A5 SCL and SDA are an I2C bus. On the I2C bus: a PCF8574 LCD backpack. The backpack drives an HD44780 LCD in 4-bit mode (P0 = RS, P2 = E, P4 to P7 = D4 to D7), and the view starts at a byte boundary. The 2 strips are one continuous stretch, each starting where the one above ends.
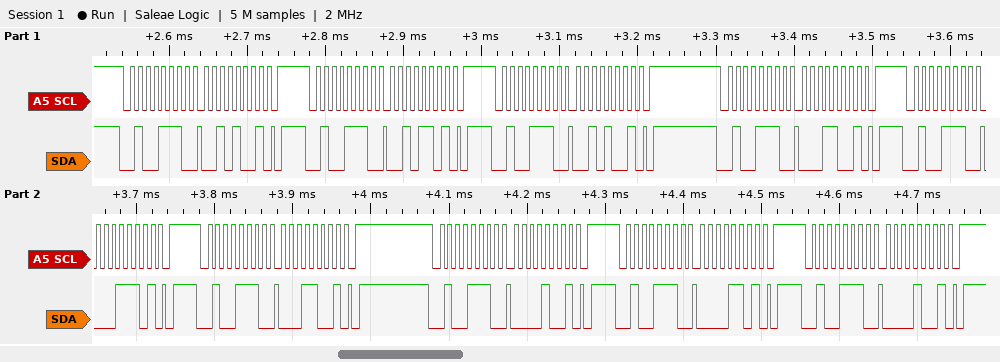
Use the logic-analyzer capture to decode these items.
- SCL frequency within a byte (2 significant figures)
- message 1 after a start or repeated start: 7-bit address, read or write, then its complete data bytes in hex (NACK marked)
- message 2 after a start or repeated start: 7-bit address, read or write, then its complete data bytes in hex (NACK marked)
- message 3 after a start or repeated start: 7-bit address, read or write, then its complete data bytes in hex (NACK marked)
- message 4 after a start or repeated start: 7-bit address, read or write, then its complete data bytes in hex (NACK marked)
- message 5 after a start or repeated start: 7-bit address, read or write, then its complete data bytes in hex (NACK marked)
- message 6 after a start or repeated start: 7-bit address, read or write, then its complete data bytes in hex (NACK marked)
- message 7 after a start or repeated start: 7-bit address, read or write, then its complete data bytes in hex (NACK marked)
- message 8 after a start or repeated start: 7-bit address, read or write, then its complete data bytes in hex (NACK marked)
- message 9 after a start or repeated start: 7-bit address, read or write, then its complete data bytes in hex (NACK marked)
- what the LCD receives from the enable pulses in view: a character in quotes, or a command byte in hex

100 kHz
0x27 write: 29
0x27 write: 2D
0x27 write: 29
0x27 write: 19
0x27 write: 1D
0x27 write: 19
0x27 write: 09
0x27 write: 0D
0x27 write: 09
'!'
